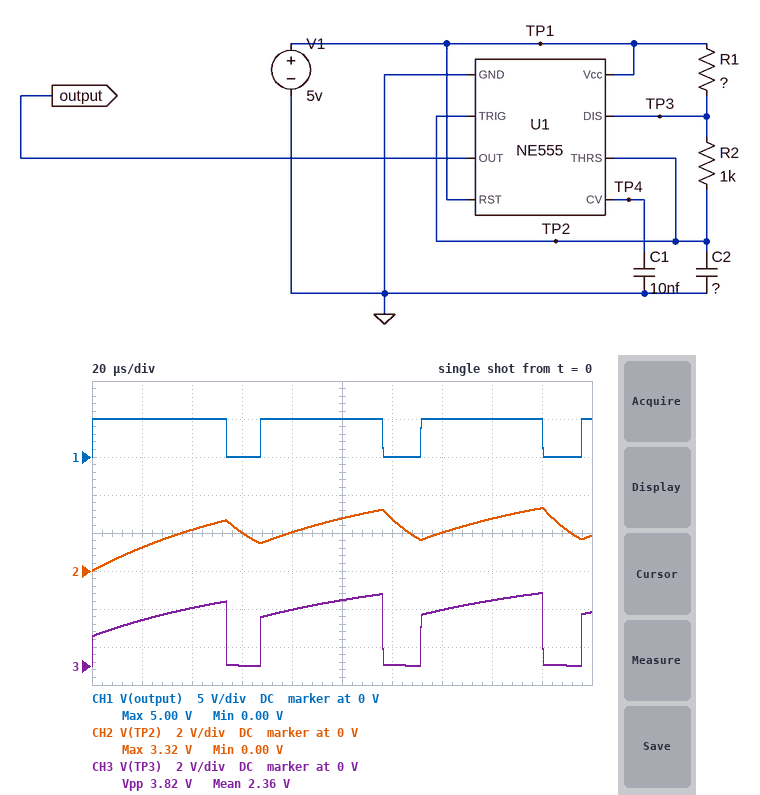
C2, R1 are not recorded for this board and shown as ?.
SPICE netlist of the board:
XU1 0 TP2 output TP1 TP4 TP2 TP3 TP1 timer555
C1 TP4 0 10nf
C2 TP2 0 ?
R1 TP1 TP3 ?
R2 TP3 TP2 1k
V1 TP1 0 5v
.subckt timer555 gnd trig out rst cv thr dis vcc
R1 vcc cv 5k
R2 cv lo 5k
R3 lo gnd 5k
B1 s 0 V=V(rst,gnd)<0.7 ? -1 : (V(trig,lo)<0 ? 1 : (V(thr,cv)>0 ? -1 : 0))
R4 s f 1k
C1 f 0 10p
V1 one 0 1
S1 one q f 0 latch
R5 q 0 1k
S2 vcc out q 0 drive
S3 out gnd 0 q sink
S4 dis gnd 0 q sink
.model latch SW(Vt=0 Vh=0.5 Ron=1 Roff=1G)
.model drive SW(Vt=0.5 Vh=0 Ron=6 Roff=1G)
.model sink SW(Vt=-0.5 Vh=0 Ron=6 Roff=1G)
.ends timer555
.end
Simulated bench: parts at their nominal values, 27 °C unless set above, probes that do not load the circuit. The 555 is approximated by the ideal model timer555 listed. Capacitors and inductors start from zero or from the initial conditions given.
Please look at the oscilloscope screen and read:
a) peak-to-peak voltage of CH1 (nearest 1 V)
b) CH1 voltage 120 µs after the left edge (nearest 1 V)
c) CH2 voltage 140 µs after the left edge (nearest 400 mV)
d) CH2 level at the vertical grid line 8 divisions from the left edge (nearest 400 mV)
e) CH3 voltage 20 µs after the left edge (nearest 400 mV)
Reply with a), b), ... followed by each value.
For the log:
a) 5 V
b) 0 V
c) 2.0 V
d) 2.8 V
e) 2.4 V
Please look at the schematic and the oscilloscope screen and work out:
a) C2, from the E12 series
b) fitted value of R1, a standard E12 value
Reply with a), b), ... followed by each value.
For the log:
a) 22 nF
b) 2.2 kΩ
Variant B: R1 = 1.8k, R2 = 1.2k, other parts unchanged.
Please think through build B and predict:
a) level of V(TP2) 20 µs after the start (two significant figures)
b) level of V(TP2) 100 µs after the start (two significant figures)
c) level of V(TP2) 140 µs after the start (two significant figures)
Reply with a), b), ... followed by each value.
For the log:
a) 1.3 V
b) 3.0 V
c) 2.4 V
